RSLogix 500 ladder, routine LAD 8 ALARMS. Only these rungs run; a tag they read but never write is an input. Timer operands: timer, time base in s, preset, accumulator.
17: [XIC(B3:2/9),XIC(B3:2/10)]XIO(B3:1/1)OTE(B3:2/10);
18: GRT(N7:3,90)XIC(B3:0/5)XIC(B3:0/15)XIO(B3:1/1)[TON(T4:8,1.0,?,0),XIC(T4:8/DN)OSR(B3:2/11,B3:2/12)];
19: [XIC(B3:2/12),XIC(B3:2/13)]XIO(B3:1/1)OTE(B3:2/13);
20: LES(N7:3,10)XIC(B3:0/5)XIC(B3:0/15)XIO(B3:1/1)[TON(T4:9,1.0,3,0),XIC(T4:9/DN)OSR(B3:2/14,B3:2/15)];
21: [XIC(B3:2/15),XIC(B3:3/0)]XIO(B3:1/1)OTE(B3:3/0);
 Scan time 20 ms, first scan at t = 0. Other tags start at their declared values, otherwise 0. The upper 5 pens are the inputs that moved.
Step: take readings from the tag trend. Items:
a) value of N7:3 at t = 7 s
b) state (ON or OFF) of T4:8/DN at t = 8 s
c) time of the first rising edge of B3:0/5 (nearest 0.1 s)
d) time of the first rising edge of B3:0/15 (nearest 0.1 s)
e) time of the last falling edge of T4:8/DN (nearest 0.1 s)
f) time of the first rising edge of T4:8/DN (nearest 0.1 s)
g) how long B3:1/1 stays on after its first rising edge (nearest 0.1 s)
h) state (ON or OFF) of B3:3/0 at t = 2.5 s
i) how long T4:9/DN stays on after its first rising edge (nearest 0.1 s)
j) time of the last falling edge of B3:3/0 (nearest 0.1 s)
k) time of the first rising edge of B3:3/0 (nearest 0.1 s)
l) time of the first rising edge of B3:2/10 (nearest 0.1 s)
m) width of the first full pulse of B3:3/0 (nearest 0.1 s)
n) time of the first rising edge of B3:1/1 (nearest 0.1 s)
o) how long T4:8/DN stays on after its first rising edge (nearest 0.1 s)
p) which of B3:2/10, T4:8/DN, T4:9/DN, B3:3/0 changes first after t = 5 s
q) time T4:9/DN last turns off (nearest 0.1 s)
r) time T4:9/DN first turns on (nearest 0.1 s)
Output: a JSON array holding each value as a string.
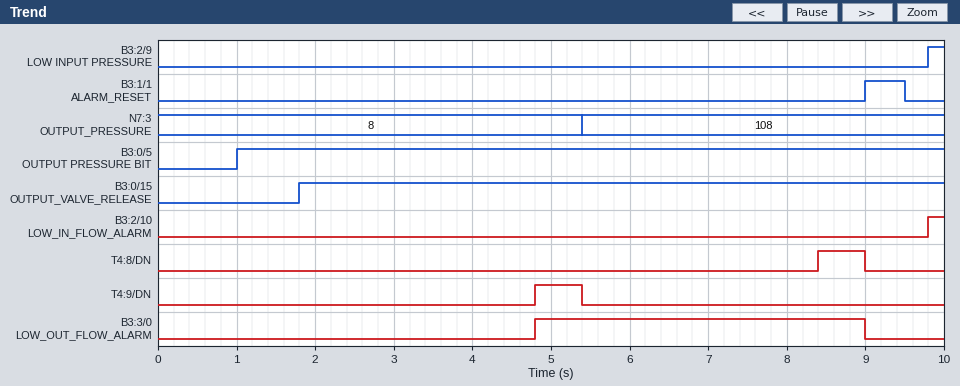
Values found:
["108", "OFF", "1.0 s", "1.8 s", "9.0 s", "8.4 s", "0.5 s", "OFF", "0.6 s", "9.0 s", "4.8 s", "9.8 s", "4.2 s", "9.0 s", "0.6 s", "T4:9/DN", "5.4 s", "4.8 s"]
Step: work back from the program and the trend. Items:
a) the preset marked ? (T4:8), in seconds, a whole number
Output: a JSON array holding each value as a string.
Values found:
["3 s"]
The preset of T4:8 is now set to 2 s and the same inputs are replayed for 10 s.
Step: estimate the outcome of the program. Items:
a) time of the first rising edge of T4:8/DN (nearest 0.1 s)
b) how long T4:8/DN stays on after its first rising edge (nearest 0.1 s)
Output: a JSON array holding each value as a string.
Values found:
["7.4 s", "1.6 s"]
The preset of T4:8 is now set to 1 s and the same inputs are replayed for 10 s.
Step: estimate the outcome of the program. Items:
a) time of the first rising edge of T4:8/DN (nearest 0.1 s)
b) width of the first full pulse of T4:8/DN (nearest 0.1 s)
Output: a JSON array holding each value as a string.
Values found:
["6.4 s", "2.6 s"]
